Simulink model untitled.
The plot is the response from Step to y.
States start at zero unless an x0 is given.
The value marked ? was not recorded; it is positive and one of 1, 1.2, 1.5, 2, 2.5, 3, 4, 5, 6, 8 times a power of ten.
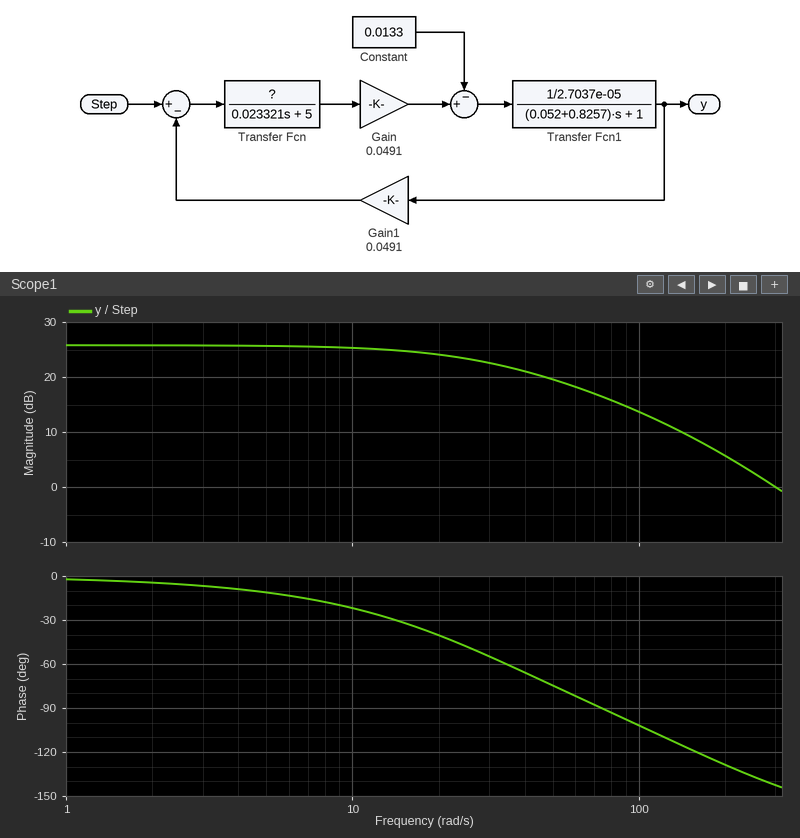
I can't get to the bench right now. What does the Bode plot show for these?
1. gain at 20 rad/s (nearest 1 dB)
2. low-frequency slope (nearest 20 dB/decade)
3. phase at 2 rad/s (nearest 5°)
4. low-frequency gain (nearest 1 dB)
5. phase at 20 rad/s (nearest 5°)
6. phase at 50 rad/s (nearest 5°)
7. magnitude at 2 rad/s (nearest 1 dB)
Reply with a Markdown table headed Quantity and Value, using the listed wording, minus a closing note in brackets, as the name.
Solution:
| Quantity | Value |
|---|---|
| gain at 20 rad/s | 24 dB |
| low-frequency slope | 0 dB/decade |
| phase at 2 rad/s | -5° |
| low-frequency gain | 26 dB |
| phase at 20 rad/s | -40° |
| phase at 50 rad/s | -75° |
| magnitude at 2 rad/s | 26 dB |
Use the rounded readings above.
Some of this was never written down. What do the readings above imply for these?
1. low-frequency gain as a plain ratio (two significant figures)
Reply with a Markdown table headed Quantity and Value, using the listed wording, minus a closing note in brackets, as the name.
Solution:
| Quantity | Value |
|---|---|
| low-frequency gain as a plain ratio | 20 |
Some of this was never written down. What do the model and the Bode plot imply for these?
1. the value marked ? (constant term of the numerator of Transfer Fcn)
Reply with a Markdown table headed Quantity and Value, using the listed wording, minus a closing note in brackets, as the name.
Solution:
| Quantity | Value |
|---|---|
| the value marked ? | 1.2 |
